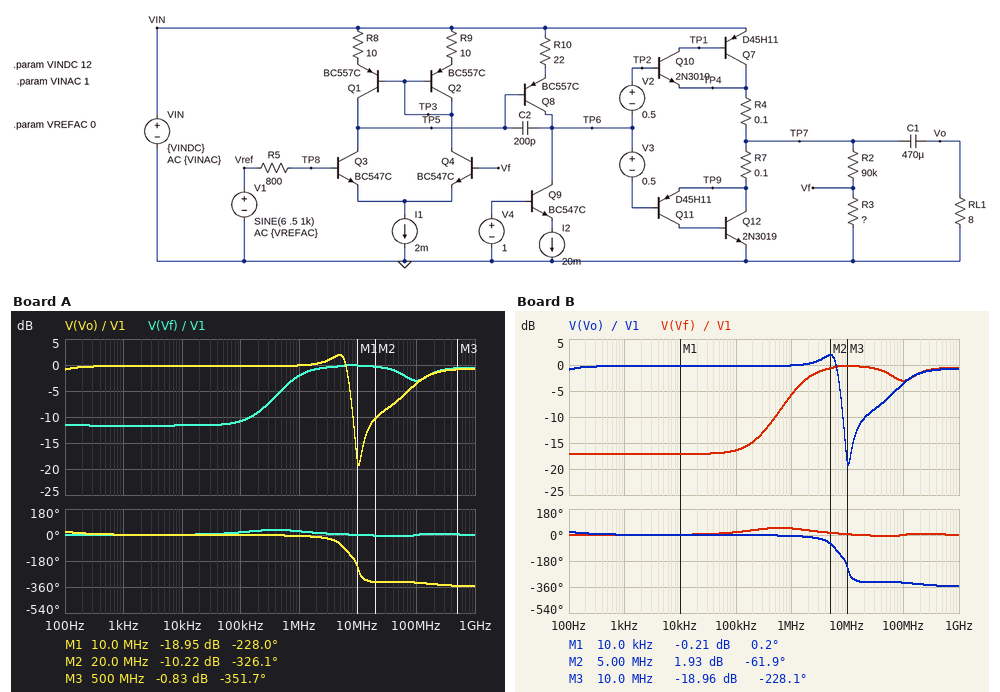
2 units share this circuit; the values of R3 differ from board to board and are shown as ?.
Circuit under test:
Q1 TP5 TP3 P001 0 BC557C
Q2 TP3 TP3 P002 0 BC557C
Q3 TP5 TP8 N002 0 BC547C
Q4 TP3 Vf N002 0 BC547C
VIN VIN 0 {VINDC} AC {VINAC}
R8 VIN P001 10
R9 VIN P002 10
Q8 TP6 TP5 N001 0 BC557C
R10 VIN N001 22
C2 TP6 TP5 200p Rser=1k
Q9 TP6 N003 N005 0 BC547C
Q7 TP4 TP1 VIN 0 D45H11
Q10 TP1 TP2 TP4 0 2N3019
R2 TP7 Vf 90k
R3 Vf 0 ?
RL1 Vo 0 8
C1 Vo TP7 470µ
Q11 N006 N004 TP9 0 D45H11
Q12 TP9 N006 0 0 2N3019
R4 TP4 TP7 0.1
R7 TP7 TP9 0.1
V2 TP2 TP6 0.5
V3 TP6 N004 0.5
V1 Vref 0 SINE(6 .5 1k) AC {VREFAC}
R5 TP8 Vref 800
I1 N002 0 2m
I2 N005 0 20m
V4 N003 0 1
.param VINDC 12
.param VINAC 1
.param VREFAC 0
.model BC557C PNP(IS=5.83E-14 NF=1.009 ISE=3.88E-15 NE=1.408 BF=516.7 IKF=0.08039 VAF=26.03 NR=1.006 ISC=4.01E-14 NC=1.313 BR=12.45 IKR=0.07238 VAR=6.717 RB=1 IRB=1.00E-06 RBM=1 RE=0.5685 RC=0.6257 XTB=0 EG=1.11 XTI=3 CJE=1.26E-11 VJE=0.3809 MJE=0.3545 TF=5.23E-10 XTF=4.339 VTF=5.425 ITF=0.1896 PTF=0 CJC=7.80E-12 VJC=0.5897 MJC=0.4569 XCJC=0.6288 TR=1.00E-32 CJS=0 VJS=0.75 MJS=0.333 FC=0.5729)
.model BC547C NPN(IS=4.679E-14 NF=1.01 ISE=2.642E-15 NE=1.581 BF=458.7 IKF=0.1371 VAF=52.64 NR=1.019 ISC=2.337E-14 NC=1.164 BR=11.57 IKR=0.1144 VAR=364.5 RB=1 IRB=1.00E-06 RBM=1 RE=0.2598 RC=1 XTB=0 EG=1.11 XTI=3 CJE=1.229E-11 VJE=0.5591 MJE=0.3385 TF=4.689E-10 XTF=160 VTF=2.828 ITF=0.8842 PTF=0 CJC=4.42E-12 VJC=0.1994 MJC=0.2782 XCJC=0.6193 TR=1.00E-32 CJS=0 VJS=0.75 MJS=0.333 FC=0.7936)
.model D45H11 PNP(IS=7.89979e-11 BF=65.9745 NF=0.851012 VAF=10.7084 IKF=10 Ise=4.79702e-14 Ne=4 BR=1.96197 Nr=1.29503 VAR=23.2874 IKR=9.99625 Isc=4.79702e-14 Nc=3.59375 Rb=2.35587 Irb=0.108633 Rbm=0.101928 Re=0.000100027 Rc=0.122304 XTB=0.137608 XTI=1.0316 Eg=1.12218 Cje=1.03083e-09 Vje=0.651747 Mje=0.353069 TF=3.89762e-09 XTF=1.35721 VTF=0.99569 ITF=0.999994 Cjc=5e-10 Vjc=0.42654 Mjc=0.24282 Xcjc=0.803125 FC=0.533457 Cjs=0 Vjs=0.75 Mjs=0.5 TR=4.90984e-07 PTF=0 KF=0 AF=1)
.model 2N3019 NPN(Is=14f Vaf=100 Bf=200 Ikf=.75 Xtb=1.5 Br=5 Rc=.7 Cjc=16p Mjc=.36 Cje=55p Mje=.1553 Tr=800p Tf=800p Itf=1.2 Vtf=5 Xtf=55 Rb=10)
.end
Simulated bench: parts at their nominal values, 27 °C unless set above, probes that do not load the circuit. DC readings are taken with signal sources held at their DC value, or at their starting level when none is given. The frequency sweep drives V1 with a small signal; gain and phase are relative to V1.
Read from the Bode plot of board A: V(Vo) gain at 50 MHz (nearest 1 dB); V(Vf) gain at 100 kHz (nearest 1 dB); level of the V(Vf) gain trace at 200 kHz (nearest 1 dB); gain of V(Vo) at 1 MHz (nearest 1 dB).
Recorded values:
-7 dB
-11 dB
-9 dB
0 dB
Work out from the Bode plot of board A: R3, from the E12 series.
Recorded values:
33 kΩ
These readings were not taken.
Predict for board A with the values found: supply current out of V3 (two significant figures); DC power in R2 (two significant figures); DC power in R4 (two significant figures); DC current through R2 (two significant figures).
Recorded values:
3.5 µA
760 µW
800 µW
92 µA
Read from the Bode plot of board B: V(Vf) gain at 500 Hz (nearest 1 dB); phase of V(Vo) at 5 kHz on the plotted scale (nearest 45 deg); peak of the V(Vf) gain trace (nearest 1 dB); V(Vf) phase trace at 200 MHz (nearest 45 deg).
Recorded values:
-17 dB
0 deg
0 dB
0 deg
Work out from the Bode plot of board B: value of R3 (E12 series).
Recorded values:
15 kΩ
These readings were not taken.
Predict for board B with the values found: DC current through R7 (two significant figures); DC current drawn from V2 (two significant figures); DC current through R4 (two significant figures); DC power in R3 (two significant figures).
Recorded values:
90 mA
6.8 µA
90 mA
170 µW
